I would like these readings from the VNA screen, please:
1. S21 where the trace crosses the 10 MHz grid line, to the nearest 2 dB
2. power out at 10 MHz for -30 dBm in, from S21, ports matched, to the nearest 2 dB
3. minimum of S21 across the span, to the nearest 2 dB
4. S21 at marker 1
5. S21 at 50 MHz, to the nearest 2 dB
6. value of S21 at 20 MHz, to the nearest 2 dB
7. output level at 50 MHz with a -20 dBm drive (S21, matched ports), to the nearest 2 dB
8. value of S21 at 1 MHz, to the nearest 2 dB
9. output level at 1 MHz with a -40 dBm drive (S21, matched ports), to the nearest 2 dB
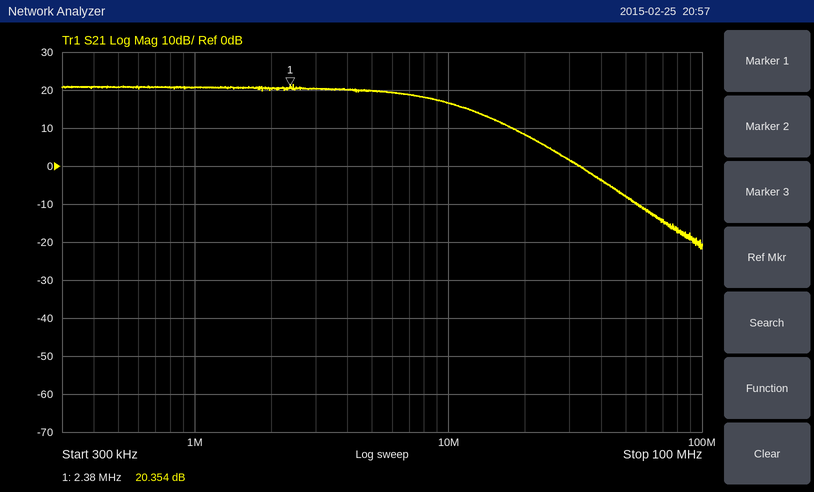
16 dB
-14 dBm
-22 dB
20.354 dB
-8 dB
8 dB
-28 dBm
20 dB
-20 dBm
